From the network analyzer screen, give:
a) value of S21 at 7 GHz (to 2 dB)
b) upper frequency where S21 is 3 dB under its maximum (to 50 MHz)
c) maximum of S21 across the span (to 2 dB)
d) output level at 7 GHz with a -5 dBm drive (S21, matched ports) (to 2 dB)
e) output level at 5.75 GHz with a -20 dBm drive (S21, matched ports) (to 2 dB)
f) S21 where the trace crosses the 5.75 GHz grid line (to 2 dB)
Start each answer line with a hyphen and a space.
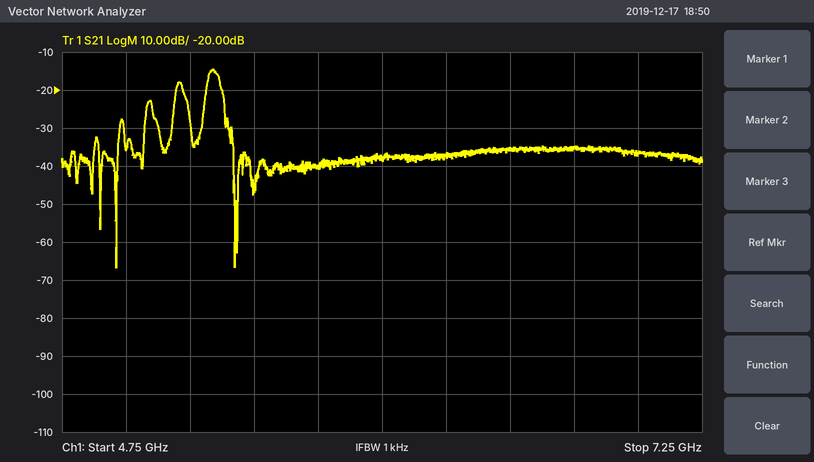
- -36 dB
- 5.35 GHz
- -14 dB
- -42 dBm
- -60 dBm
- -40 dB
